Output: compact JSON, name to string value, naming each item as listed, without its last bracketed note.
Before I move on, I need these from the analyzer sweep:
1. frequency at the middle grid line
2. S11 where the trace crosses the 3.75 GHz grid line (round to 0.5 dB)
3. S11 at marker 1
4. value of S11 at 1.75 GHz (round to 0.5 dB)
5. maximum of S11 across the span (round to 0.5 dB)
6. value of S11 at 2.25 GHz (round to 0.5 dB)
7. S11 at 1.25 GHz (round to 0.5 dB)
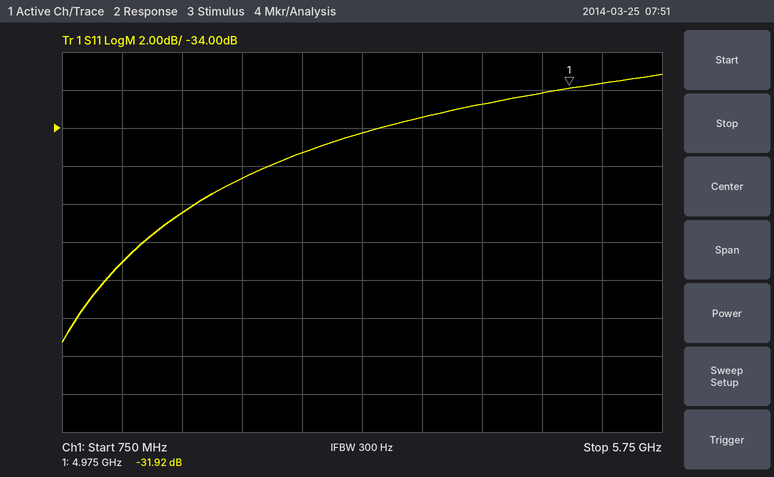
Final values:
{"frequency at the middle grid line": "3.25 GHz", "S11 where the trace crosses the 3.75 GHz grid line": "-33.5 dB", "S11 at marker 1": "-31.92 dB", "value of S11 at 1.75 GHz": "-38.5 dB", "maximum of S11 across the span": "-31.0 dB", "value of S11 at 2.25 GHz": "-36.5 dB", "S11 at 1.25 GHz": "-41.0 dB"}
